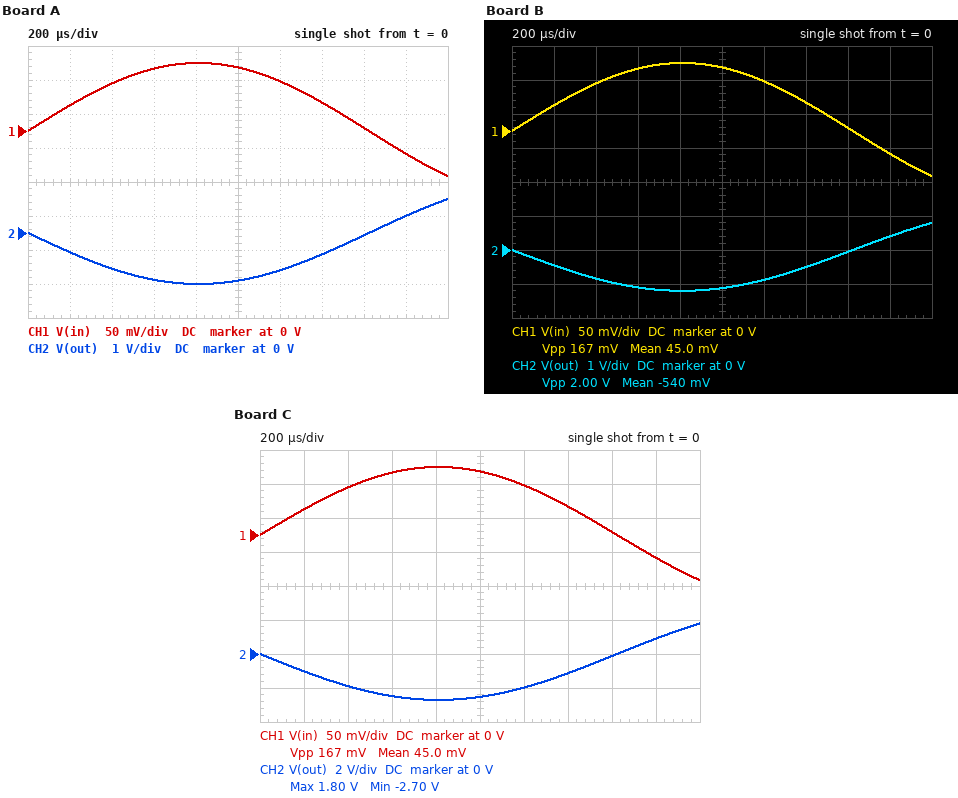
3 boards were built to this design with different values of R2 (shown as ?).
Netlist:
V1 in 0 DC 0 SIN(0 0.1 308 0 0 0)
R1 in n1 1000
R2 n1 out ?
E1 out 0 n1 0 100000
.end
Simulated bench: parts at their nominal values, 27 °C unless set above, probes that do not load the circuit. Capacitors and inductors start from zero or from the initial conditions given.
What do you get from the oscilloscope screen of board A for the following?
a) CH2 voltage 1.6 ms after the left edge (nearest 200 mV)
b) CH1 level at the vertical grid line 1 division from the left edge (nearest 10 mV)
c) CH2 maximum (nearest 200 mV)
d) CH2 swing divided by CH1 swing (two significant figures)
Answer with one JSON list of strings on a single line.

["0 V", "40 mV", "1.0 V", "15"]
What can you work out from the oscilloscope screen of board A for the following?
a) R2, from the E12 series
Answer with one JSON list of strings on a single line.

["15 kΩ"]
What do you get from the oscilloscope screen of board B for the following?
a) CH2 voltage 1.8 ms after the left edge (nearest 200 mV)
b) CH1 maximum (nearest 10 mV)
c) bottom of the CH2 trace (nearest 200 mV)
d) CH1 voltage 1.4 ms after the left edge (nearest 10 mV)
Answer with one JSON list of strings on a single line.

["400 mV", "100 mV", "-1.2 V", "40 mV"]
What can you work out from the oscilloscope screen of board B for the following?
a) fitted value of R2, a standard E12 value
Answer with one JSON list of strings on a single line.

["12 kΩ"]
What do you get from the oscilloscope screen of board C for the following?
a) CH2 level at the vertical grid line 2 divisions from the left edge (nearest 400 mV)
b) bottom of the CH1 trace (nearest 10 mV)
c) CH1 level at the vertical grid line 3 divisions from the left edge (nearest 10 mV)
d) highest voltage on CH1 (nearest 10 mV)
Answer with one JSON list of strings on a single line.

["-2.0 V", "-70 mV", "90 mV", "100 mV"]
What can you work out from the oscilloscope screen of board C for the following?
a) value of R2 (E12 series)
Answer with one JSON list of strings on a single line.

["27 kΩ"]
